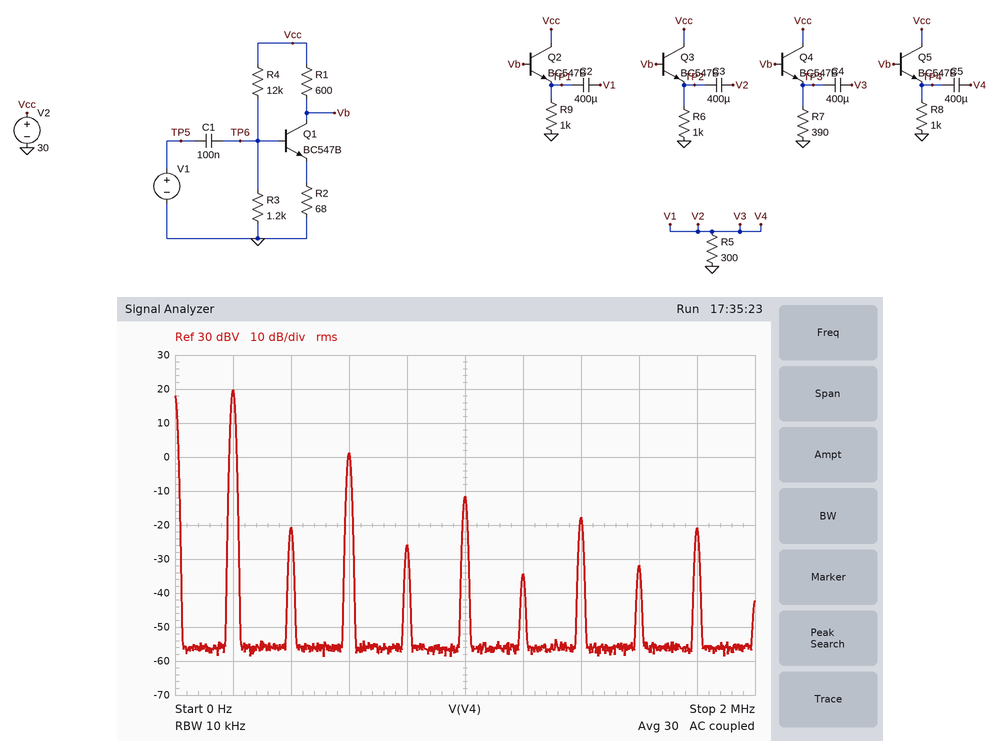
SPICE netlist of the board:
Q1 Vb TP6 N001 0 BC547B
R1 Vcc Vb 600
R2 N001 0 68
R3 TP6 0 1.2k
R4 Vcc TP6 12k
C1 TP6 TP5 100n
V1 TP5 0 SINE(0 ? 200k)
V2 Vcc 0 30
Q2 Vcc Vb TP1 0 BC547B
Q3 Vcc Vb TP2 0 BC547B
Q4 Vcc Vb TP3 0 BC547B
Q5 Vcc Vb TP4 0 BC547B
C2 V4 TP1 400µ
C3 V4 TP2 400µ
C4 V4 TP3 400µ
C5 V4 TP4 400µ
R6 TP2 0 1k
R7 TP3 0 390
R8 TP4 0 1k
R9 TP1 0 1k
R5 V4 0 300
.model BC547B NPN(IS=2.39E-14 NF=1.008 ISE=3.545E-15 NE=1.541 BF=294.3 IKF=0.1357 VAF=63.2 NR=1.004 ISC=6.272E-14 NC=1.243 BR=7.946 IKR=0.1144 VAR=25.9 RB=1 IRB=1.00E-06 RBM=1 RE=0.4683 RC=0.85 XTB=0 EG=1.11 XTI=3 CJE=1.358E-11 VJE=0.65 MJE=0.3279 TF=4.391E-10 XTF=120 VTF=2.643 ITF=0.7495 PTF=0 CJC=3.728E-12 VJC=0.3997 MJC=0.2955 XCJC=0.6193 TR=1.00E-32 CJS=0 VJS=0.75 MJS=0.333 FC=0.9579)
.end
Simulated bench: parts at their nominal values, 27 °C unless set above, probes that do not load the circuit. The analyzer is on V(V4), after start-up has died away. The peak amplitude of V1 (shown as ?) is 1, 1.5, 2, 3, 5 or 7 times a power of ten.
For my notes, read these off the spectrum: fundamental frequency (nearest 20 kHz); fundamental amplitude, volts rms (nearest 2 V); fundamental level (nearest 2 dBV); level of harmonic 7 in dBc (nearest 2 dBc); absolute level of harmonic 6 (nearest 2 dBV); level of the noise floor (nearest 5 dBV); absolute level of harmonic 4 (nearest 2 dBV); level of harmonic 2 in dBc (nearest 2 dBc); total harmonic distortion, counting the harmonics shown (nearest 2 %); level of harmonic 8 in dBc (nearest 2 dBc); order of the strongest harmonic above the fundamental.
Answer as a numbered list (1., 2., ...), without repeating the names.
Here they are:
1. 200 kHz
2. 10 V
3. 20 dBV
4. -38 dBc
5. -34 dBV
6. -55 dBV
7. -26 dBV
8. -40 dBc
9. 12 %
10. -52 dBc
11. 3
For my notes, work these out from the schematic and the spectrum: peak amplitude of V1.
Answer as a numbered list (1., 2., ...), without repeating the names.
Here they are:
1. 2 V
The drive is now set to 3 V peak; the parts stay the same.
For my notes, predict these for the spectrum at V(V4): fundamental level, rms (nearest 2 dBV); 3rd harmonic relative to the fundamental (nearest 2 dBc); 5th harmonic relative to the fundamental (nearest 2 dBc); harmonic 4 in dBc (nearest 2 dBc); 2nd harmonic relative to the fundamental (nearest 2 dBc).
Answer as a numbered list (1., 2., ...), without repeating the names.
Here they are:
1. 20 dBV
2. -16 dBc
3. -36 dBc
4. -20 dBc
5. -14 dBc
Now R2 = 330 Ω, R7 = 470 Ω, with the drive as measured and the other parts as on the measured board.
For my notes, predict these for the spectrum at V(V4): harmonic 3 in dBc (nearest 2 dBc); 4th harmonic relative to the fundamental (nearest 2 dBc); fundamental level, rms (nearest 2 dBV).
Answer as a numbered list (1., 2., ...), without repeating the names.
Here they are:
1. -48 dBc
2. -56 dBc
3. 8 dBV
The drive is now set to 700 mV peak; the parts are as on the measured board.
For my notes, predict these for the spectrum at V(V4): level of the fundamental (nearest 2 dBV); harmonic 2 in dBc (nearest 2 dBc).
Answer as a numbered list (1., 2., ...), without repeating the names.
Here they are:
1. 12 dBV
2. -58 dBc
